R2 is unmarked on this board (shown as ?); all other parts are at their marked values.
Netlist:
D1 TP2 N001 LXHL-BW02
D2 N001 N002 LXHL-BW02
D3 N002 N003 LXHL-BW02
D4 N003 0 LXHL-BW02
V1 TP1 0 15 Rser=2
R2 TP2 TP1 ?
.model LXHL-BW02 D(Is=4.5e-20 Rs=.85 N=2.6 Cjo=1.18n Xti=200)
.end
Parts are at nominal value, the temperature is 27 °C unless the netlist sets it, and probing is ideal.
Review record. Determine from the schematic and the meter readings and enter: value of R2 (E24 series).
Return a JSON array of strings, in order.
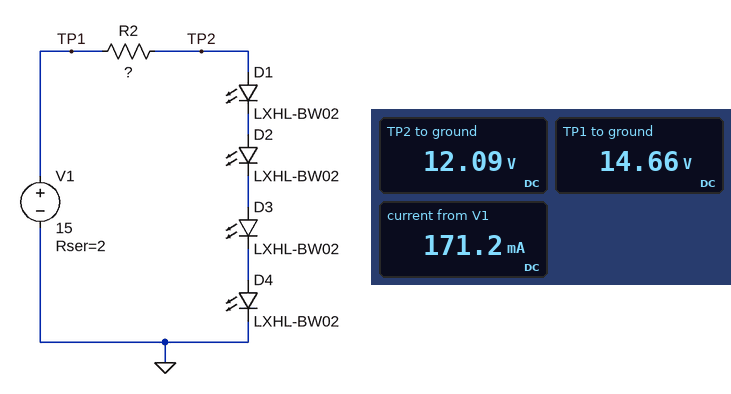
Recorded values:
["15 Ω"]
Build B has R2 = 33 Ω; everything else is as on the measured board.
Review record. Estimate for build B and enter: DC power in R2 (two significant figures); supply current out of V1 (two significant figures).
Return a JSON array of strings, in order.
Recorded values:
["300 mW", "95 mA"]
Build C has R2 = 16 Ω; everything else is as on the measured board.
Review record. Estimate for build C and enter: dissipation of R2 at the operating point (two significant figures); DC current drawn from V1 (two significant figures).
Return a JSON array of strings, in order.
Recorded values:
["430 mW", "160 mA"]
